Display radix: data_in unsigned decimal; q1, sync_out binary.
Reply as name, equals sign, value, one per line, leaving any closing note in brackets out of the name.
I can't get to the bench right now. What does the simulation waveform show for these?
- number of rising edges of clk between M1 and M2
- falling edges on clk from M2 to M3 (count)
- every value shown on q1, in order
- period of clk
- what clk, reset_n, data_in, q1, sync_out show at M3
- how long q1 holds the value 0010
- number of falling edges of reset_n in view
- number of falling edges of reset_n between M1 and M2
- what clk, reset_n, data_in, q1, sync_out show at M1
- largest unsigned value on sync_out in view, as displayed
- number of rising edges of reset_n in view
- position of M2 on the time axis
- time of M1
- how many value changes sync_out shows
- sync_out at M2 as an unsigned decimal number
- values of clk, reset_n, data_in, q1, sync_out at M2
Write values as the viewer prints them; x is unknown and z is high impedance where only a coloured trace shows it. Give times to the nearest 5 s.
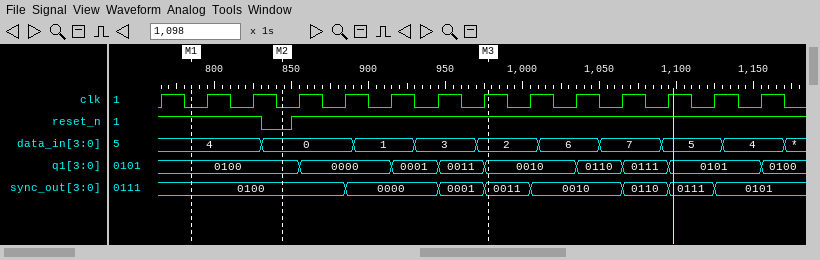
number of rising edges of clk between M1 and M2 = 2
falling edges on clk from M2 to M3 = 4
every value shown on q1, in order = 0100, 0000, 0001, 0011, 0010, 0110, 0111, 0101, 0100
period of clk = 30 s
what clk, reset_n, data_in, q1, sync_out show at M3 = clk=1, reset_n=1, data_in=2, q1=0010, sync_out=0011
how long q1 holds the value 0010 = 60 s
number of falling edges of reset_n in view = 1
number of falling edges of reset_n between M1 and M2 = 1
what clk, reset_n, data_in, q1, sync_out show at M1 = clk=0, reset_n=1, data_in=4, q1=0100, sync_out=0100
largest unsigned value on sync_out in view, as displayed = 0111
number of rising edges of reset_n in view = 1
position of M2 on the time axis = 845 s
time of M1 = 785 s
how many value changes sync_out shows = 7
sync_out at M2 as an unsigned decimal number = 4
values of clk, reset_n, data_in, q1, sync_out at M2 = clk=0, reset_n=0, data_in=0, q1=0100, sync_out=0100
